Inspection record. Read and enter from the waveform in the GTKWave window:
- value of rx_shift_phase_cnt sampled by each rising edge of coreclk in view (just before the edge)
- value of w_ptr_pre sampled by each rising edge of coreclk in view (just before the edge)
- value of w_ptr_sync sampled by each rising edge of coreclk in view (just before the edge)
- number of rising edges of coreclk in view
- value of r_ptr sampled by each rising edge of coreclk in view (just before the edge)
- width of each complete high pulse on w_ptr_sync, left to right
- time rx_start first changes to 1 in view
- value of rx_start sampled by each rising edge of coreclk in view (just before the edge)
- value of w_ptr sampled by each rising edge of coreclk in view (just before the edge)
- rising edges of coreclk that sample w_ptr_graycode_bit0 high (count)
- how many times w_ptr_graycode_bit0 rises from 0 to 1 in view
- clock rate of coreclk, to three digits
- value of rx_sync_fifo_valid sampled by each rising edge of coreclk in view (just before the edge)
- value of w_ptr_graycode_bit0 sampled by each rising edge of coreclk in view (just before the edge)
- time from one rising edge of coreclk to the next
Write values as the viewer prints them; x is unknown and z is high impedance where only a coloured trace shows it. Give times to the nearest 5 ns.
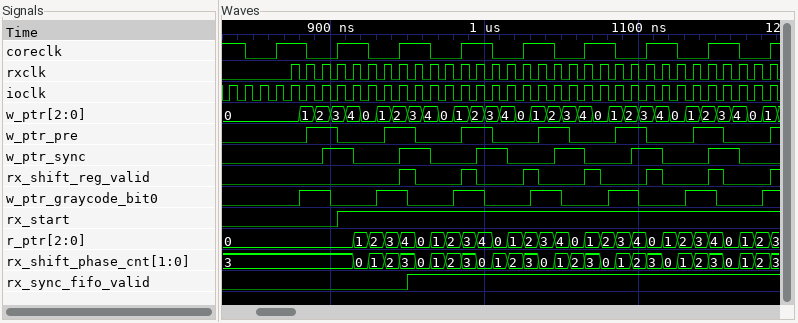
3, 3, 2, 2, 2, 2, 2, 2, 2
0 1 1 0 0 0 1 1 0
0 1 0 0 0 1 1 0 0
9
0, 0, 3, 2, 1, 0, 4, 3, 2
20 ns, 20 ns, 20 ns, 20 ns, 20 ns, 20 ns
905 ns
0 0 1 1 1 1 1 1 1
0, 3, 2, 1, 0, 4, 3, 2, 1
4
7
25.0 MHz
0 0 0 1 1 1 1 1 1
0 0 1 1 0 0 0 1 1
40 ns
